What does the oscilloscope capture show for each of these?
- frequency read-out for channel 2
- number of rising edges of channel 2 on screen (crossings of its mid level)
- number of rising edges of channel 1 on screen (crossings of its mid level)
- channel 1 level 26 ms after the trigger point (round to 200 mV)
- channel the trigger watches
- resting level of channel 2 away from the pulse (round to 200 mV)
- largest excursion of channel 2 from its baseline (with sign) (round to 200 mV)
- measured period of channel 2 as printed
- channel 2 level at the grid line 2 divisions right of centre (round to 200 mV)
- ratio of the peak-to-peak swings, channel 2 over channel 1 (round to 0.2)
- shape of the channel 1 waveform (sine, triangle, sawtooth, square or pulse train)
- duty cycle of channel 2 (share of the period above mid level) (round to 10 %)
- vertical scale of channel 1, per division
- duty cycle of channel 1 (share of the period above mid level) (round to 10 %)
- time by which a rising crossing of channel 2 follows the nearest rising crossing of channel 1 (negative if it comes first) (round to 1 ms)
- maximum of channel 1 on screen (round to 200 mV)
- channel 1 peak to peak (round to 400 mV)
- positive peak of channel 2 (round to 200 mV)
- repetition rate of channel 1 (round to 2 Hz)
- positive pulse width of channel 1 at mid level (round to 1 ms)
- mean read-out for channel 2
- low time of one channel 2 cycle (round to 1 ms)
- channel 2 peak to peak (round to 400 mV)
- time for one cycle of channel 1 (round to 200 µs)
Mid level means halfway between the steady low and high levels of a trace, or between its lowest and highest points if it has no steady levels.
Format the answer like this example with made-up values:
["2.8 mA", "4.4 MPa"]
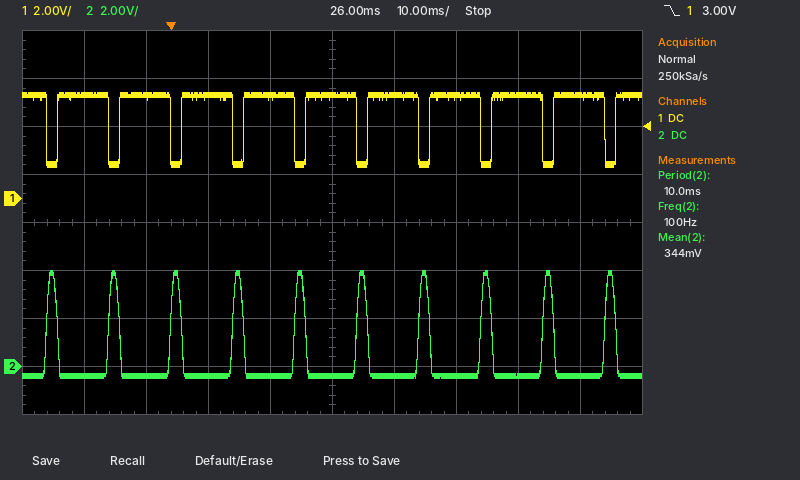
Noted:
["100 Hz", "10", "10", "4.2 V", "channel 1", "-400 mV", "+4.4 V", "10.0 ms", "-400 mV", "1.4", "pulse train", "20 %", "2 V", "80 %", "-2 ms", "4.4 V", "3.2 V", "4.0 V", "100 Hz", "8 ms", "344 mV", "8 ms", "4.4 V", "10.0 ms"]
